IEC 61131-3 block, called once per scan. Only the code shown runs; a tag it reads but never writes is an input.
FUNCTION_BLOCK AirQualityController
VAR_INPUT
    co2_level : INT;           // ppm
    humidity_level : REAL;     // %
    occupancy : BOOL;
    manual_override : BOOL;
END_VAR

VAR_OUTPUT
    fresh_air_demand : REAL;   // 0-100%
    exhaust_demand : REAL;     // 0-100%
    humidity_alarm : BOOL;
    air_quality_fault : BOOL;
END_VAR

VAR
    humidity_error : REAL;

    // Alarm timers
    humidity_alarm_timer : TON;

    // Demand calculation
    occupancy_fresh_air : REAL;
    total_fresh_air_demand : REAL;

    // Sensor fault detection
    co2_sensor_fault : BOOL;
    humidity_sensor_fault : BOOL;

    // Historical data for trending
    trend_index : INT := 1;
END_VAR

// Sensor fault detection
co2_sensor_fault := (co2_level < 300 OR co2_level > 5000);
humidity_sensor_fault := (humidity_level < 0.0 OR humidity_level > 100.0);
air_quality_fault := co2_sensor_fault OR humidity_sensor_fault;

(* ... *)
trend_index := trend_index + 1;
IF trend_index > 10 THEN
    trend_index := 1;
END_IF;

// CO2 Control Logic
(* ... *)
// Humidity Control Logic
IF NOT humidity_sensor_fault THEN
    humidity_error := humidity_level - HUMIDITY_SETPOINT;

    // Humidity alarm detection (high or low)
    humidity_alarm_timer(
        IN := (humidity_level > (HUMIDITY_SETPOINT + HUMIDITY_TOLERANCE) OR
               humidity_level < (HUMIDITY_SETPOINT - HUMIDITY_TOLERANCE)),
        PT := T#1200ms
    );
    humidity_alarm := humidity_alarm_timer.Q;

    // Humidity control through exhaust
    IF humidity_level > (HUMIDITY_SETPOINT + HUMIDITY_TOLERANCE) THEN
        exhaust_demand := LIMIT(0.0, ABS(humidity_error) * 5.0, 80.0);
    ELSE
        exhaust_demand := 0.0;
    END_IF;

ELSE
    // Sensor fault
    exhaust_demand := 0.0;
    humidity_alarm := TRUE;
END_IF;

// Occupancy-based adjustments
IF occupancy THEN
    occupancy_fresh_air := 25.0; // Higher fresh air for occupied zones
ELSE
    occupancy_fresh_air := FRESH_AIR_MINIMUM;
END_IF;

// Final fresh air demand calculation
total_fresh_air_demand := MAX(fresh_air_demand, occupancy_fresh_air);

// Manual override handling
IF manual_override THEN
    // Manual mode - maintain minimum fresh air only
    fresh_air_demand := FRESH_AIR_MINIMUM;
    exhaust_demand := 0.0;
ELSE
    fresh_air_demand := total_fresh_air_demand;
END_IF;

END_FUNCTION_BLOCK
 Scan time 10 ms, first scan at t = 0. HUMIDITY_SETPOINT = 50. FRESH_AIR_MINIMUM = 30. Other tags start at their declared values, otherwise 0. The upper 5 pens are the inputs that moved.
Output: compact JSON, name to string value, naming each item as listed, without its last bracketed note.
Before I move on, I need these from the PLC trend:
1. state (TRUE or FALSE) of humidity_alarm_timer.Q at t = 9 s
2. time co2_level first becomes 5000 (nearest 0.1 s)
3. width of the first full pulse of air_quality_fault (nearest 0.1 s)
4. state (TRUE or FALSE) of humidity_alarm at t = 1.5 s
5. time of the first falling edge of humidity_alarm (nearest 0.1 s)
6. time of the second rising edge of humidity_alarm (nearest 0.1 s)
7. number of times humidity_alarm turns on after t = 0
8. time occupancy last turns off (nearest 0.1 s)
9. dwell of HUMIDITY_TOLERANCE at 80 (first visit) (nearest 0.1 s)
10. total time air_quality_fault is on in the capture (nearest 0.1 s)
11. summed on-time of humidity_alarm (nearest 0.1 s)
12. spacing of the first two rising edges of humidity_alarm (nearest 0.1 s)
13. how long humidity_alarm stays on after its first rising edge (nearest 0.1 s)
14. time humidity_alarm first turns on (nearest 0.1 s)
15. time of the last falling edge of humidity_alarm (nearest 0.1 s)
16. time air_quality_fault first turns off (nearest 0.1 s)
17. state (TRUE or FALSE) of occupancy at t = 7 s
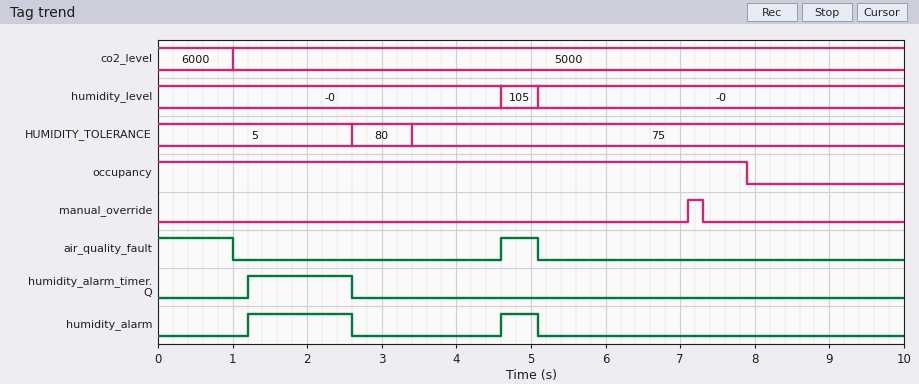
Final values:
{"state (TRUE or FALSE) of humidity_alarm_timer.Q at t = 9 s": "FALSE", "time co2_level first becomes 5000": "1.0 s", "width of the first full pulse of air_quality_fault": "0.5 s", "state (TRUE or FALSE) of humidity_alarm at t = 1.5 s": "TRUE", "time of the first falling edge of humidity_alarm": "2.6 s", "time of the second rising edge of humidity_alarm": "4.6 s", "number of times humidity_alarm turns on after t = 0": "2", "time occupancy last turns off": "7.9 s", "dwell of HUMIDITY_TOLERANCE at 80 (first visit)": "0.8 s", "total time air_quality_fault is on in the capture": "1.5 s", "summed on-time of humidity_alarm": "1.9 s", "spacing of the first two rising edges of humidity_alarm": "3.4 s", "how long humidity_alarm stays on after its first rising edge": "1.4 s", "time humidity_alarm first turns on": "1.2 s", "time of the last falling edge of humidity_alarm": "5.1 s", "time air_quality_fault first turns off": "1.0 s", "state (TRUE or FALSE) of occupancy at t = 7 s": "TRUE"}
